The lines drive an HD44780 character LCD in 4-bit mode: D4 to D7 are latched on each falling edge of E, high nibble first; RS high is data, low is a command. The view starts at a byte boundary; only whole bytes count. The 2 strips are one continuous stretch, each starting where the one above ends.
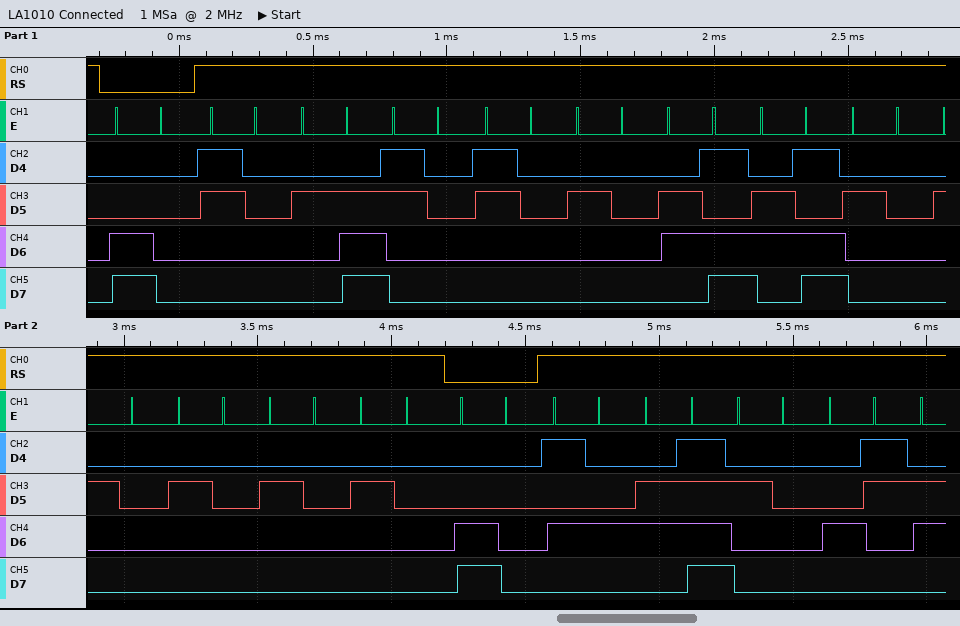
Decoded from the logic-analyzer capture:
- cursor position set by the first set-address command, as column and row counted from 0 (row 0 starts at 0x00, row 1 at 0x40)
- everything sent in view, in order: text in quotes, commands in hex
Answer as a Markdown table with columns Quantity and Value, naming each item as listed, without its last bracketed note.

| Quantity | Value |
|---|---|
| cursor position set by the first set-address command, as column and row counted from 0 | column 0, row 1 |
| everything sent in view, in order: text in quotes, commands in hex | 0xC0 "0.00 mm     " 0xC0 "To C" |
